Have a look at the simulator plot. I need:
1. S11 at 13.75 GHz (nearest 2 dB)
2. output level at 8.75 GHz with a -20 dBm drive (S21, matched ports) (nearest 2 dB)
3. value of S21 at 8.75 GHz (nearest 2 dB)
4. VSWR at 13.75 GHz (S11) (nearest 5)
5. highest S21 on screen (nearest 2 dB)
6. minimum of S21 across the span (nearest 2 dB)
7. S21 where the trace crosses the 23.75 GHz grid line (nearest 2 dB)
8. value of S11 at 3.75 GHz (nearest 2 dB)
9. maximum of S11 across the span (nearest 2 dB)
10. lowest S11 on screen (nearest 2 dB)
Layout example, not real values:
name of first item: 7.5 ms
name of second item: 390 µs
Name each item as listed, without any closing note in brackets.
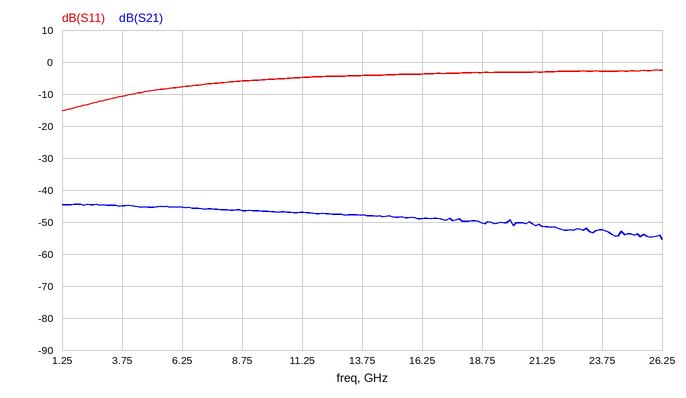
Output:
S11 at 13.75 GHz: -4 dB
output level at 8.75 GHz with a -20 dBm drive (S21, matched ports): -66 dBm
value of S21 at 8.75 GHz: -46 dB
VSWR at 13.75 GHz (S11): 5
highest S21 on screen: -44 dB
minimum of S21 across the span: -56 dB
S21 where the trace crosses the 23.75 GHz grid line: -52 dB
value of S11 at 3.75 GHz: -10 dB
maximum of S11 across the span: -2 dB
lowest S11 on screen: -16 dB
